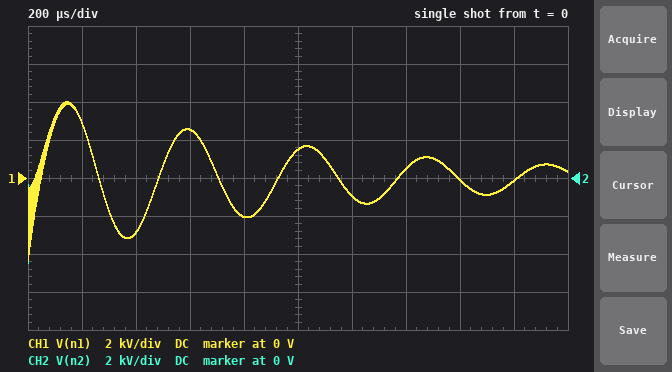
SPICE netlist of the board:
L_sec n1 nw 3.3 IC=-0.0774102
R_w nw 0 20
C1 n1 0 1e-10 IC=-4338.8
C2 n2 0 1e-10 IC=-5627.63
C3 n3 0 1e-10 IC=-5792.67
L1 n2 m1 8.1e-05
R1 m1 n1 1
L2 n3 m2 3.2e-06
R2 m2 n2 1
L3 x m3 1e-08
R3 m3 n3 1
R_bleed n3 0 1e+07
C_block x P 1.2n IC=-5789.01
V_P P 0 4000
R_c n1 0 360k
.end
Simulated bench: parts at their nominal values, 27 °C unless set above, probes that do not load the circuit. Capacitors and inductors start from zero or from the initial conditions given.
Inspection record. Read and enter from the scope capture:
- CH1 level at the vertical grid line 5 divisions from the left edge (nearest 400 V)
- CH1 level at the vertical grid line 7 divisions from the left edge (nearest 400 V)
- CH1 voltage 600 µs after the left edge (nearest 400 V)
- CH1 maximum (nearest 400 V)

1.6 kV
400 V
2.4 kV
4.0 kV
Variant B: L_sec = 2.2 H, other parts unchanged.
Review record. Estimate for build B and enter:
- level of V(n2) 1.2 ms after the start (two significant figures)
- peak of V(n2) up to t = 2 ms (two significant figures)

1.2 kV
3.5 kV
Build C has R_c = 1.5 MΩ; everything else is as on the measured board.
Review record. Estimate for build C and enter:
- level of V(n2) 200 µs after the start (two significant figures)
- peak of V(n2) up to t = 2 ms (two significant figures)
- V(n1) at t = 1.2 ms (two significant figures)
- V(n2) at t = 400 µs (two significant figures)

3.3 kV
4.3 kV
-2.2 kV
-3.7 kV
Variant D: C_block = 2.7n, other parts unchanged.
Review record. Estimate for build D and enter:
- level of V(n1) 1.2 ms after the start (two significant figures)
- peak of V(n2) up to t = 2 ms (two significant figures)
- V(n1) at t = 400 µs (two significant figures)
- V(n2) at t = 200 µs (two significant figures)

-1.8 kV
3.1 kV
-560 V
3.0 kV
